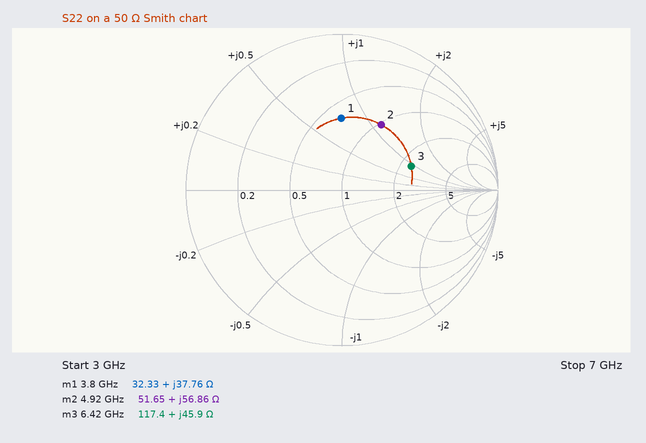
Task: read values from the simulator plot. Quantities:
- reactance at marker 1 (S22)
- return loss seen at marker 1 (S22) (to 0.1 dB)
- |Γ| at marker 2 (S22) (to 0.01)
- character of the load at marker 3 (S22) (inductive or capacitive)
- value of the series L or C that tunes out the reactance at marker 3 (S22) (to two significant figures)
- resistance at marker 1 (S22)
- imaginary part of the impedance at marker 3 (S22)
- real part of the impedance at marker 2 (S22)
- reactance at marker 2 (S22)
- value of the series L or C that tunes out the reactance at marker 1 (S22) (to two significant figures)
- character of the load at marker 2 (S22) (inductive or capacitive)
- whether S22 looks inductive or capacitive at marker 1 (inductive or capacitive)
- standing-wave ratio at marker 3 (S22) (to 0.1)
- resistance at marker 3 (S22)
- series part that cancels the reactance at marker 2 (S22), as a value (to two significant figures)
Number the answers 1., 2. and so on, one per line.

1. +37.76 Ω
2. 6.7 dB
3. 0.49
4. inductive
5. 540 fF
6. 32.33 Ω
7. +45.9 Ω
8. 51.65 Ω
9. +56.86 Ω
10. 1.1 pF
11. inductive
12. inductive
13. 2.8
14. 117.4 Ω
15. 570 fF
